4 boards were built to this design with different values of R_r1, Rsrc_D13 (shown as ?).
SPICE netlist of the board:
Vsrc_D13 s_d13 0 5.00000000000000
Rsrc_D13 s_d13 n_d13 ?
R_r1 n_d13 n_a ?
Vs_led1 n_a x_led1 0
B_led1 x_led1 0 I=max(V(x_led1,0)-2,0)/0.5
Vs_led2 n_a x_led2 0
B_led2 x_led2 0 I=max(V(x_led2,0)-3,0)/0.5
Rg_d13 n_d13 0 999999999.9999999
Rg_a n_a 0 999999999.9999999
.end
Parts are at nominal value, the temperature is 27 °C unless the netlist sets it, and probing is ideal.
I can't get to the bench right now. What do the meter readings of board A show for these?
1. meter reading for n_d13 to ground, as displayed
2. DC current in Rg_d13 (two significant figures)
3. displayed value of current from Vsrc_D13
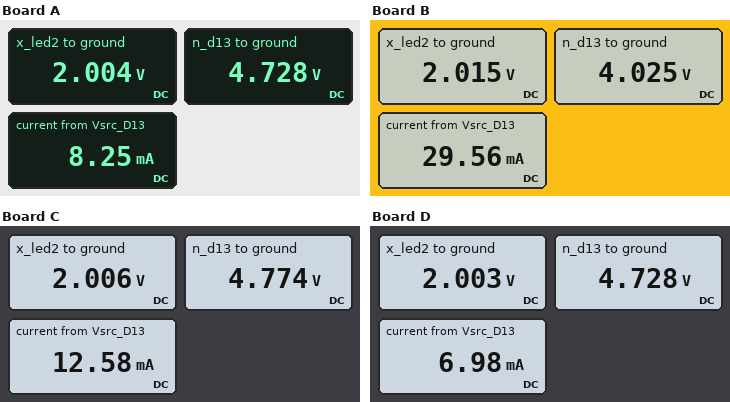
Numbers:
4.728 V
4.7 nA
8.25 mA
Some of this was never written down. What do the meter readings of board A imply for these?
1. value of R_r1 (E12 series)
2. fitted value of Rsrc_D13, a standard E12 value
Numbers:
330 Ω
33 Ω
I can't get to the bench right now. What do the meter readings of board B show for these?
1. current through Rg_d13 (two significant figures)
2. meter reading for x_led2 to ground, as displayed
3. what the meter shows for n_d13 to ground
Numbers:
4.0 nA
2.015 V
4.025 V
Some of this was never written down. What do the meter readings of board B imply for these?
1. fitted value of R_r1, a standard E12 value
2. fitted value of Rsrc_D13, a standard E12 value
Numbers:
68 Ω
33 Ω
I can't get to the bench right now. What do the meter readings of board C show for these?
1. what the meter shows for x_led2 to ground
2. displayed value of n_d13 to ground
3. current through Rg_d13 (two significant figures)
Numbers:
2.006 V
4.774 V
4.8 nA
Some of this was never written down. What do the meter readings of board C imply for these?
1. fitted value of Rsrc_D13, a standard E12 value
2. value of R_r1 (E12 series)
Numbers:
18 Ω
220 Ω
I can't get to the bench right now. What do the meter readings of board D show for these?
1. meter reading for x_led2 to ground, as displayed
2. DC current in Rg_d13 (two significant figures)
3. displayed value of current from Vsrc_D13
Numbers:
2.003 V
4.7 nA
6.98 mA
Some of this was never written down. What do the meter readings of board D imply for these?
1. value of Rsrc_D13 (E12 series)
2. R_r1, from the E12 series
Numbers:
39 Ω
390 Ω
